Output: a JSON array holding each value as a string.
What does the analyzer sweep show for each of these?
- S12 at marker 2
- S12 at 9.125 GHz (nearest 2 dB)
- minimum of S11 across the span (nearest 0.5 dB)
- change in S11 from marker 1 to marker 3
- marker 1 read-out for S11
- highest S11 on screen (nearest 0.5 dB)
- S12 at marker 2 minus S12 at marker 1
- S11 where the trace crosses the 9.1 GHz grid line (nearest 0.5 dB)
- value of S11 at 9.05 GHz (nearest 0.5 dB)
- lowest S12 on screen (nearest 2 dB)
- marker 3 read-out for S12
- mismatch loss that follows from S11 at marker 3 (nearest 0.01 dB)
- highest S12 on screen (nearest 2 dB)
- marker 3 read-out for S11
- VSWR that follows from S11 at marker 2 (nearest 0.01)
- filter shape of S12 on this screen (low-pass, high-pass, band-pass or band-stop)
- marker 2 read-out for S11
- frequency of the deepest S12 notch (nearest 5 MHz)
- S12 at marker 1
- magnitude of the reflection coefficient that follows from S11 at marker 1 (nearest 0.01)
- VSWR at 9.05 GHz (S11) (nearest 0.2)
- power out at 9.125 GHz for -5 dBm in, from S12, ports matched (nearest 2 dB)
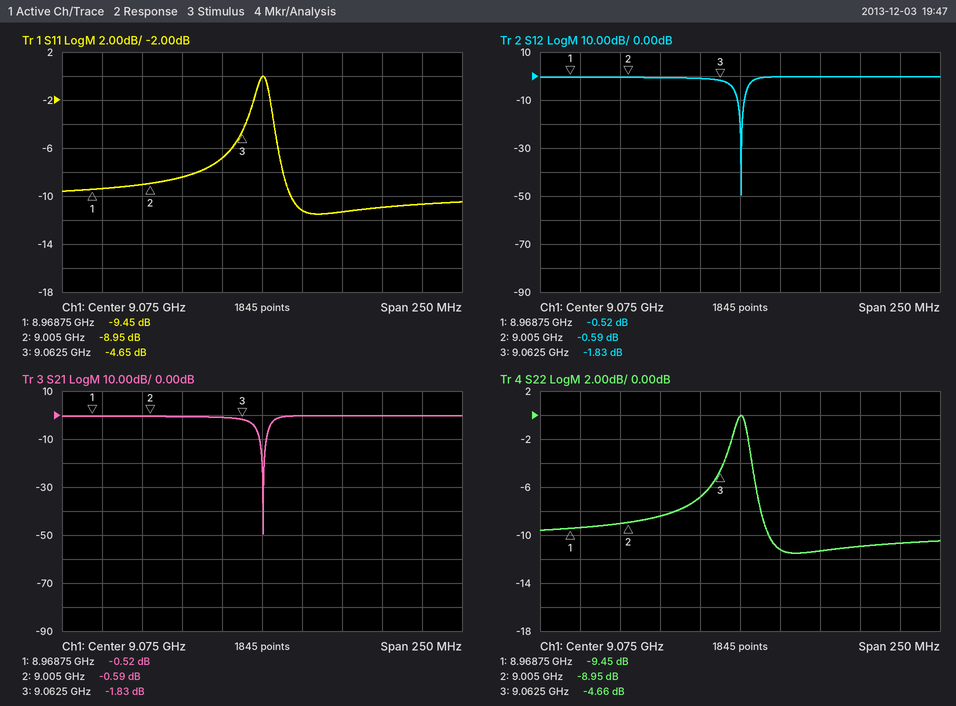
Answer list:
["-0.59 dB", "0 dB", "-11.5 dB", "4.80 dB", "-9.45 dB", "0.0 dB", "-0.07 dB", "-11.0 dB", "-7.0 dB", "-50 dB", "-1.83 dB", "1.82 dB", "0 dB", "-4.65 dB", "2.11", "band-stop", "-8.95 dB", "9.075 GHz", "-0.52 dB", "0.34", "2.6", "-6 dBm"]
